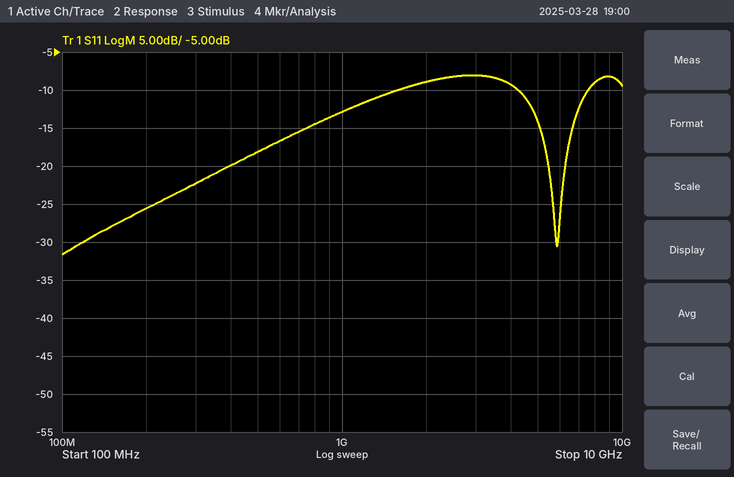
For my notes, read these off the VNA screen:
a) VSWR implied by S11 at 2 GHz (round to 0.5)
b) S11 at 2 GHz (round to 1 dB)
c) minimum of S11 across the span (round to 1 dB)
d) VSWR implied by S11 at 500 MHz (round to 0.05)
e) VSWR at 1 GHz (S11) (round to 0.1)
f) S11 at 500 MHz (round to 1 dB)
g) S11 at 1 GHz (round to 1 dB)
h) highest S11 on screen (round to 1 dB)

2.0
-9 dB
-32 dB
1.30
1.6
-18 dB
-13 dB
-8 dB
